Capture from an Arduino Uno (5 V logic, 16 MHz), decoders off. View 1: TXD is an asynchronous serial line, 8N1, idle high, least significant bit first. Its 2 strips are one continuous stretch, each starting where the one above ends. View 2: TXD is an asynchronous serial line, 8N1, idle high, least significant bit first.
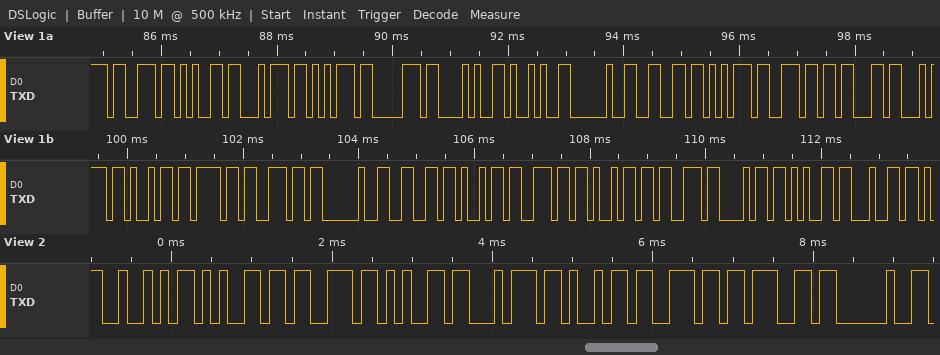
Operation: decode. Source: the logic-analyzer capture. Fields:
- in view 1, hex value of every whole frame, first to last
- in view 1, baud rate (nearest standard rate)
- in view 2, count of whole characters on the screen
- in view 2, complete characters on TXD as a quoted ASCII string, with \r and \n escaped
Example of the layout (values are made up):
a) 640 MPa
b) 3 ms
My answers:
a) 73 65 74 75 70 28 29 20 66 75 6E 63 74 69 6F 6E 20 66 69 6E 69 73 68 65 64
b) 9600 baud
c) 9
d) "Reseting "
